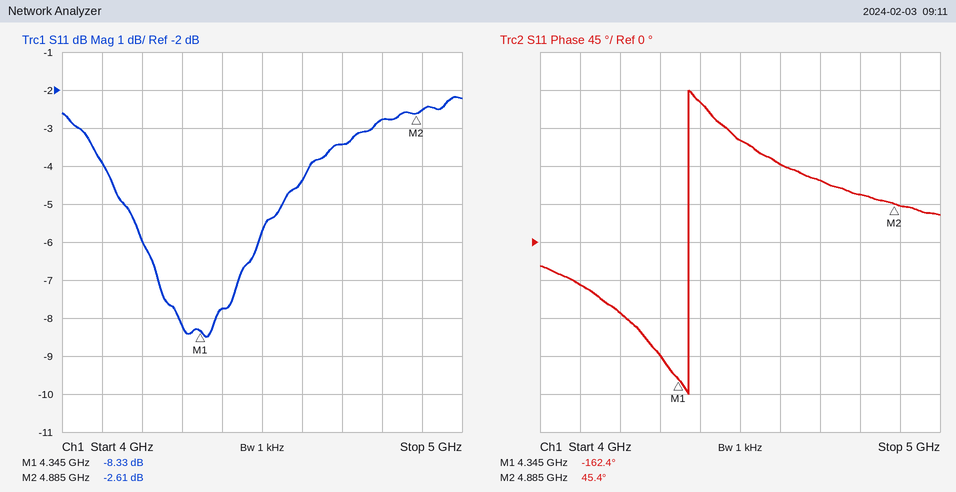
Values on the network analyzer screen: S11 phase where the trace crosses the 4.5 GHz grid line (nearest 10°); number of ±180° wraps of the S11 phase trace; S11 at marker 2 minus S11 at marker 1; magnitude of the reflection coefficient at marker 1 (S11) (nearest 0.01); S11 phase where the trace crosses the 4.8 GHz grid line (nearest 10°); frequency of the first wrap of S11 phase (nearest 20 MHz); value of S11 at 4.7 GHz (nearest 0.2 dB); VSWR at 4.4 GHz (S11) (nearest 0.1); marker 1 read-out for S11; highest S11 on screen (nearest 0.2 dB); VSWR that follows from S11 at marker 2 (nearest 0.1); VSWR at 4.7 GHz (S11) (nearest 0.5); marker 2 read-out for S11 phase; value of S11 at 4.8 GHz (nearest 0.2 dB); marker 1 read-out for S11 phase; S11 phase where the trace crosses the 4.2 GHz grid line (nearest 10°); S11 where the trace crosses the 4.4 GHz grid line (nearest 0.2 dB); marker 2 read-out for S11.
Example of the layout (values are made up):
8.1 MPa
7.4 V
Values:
120°
1
5.72 dB
0.38
60°
4.38 GHz
-3.4 dB
2.4
-8.33 dB
-2.2 dB
6.7
5.0
45.4°
-2.8 dB
-162.4°
-80°
-7.8 dB
-2.61 dB
